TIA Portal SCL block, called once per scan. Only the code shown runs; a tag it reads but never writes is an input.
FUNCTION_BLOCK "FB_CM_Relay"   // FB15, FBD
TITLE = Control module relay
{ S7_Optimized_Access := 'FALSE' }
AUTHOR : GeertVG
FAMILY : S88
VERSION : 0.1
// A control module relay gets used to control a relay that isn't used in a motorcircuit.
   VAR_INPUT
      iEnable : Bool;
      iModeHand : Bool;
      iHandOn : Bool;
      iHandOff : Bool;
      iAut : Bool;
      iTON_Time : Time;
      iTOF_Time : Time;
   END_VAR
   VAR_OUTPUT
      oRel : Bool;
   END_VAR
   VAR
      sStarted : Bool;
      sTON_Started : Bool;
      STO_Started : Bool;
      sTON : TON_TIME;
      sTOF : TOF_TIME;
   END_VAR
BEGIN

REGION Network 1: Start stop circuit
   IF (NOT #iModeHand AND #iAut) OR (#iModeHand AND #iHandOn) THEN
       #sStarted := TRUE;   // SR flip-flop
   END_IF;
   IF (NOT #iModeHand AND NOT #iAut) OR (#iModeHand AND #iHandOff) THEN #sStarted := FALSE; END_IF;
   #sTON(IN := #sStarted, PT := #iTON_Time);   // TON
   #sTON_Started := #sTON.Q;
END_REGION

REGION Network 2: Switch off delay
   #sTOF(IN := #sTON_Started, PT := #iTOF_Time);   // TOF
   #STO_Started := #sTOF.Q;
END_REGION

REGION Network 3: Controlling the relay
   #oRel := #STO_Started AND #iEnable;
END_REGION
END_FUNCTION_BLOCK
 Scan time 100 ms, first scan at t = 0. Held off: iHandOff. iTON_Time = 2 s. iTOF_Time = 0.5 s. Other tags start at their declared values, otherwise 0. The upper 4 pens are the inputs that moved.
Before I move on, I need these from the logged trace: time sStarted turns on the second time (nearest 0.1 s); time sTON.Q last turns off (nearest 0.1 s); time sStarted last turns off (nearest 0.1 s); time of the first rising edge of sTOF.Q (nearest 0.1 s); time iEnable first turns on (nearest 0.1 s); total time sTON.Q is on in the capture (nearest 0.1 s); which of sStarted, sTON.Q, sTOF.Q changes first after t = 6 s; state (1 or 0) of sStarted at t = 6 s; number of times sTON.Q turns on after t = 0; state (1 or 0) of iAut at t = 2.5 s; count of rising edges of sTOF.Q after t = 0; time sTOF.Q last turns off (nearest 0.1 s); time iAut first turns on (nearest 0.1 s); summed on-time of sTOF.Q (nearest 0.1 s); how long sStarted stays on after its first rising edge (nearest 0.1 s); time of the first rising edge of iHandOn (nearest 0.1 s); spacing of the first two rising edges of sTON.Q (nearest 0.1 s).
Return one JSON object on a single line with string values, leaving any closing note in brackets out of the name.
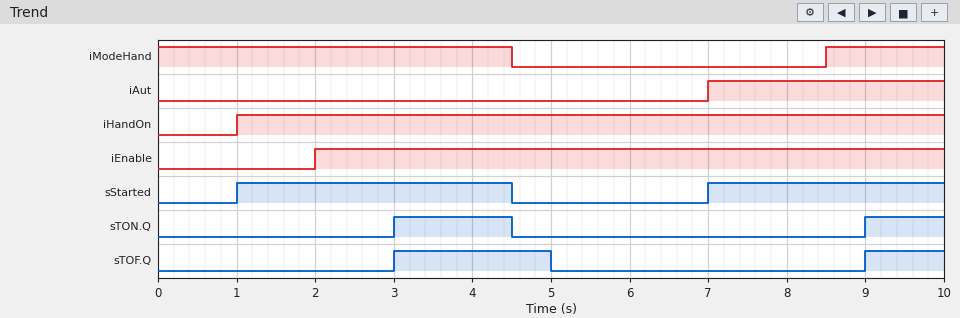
{"time sStarted turns on the second time": "7.0 s", "time sTON.Q last turns off": "4.5 s", "time sStarted last turns off": "4.5 s", "time of the first rising edge of sTOF.Q": "3.0 s", "time iEnable first turns on": "2.0 s", "total time sTON.Q is on in the capture": "2.5 s", "which of sStarted, sTON.Q, sTOF.Q changes first after t = 6 s": "sStarted", "state (1 or 0) of sStarted at t = 6 s": "0", "number of times sTON.Q turns on after t = 0": "2", "state (1 or 0) of iAut at t = 2.5 s": "0", "count of rising edges of sTOF.Q after t = 0": "2", "time sTOF.Q last turns off": "5.0 s", "time iAut first turns on": "7.0 s", "summed on-time of sTOF.Q": "3.0 s", "how long sStarted stays on after its first rising edge": "3.5 s", "time of the first rising edge of iHandOn": "1.0 s", "spacing of the first two rising edges of sTON.Q": "6.0 s"}
